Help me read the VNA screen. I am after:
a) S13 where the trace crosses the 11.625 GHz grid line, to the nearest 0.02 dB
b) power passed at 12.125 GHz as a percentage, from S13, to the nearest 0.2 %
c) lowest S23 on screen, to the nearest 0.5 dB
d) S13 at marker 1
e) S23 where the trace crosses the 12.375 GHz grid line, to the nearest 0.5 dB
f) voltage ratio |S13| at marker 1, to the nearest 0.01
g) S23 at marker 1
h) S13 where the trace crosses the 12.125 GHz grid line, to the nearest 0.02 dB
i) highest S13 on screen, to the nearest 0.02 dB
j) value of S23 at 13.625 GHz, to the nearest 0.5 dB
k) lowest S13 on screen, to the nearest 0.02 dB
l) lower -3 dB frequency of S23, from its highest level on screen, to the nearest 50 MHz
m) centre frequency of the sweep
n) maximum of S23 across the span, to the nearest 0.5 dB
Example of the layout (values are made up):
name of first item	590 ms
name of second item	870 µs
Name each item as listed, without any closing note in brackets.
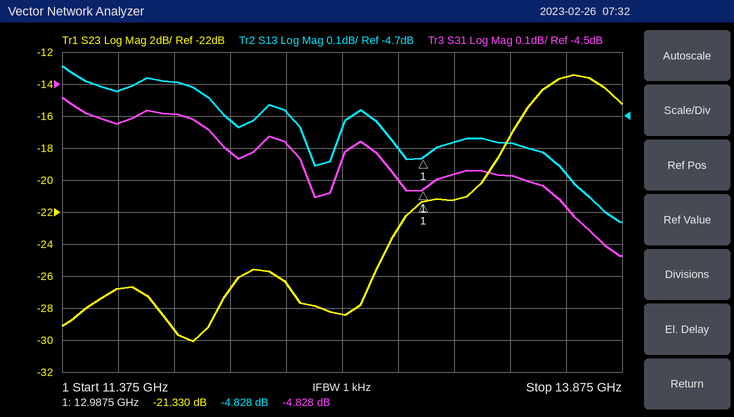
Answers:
S13 where the trace crosses the 11.625 GHz grid line, to the nearest 0.02 dB	-4.62 dB
power passed at 12.125 GHz as a percentage, from S13, to the nearest 0.2 %	33.8 %
lowest S23 on screen, to the nearest 0.5 dB	-30.0 dB
S13 at marker 1	-4.828 dB
S23 where the trace crosses the 12.375 GHz grid line, to the nearest 0.5 dB	-26.5 dB
voltage ratio |S13| at marker 1, to the nearest 0.01	0.57
S23 at marker 1	-21.330 dB
S13 where the trace crosses the 12.125 GHz grid line, to the nearest 0.02 dB	-4.72 dB
highest S13 on screen, to the nearest 0.02 dB	-4.54 dB
value of S23 at 13.625 GHz, to the nearest 0.5 dB	-13.5 dB
lowest S13 on screen, to the nearest 0.02 dB	-5.04 dB
lower -3 dB frequency of S23, from its highest level on screen, to the nearest 50 MHz	13.40 GHz
centre frequency of the sweep	12.625 GHz
maximum of S23 across the span, to the nearest 0.5 dB	-13.5 dB
